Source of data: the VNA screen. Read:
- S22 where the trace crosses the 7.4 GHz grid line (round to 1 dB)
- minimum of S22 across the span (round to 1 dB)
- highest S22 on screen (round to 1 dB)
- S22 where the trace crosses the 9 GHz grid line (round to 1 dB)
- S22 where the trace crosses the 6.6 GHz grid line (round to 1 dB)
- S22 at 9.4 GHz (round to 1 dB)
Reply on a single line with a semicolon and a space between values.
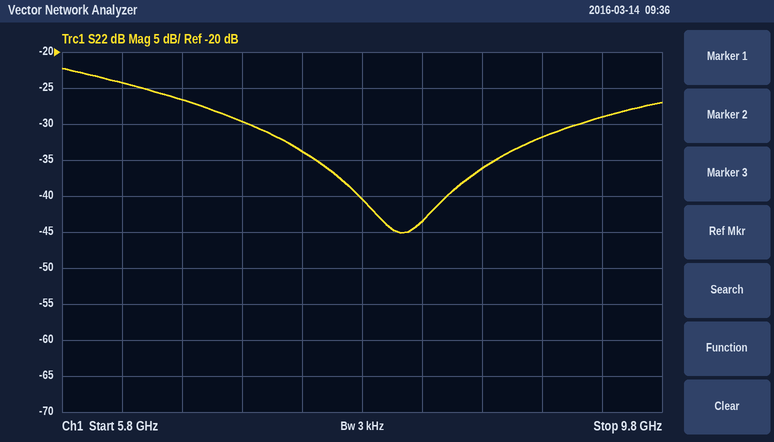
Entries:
-34 dB; -45 dB; -22 dB; -32 dB; -27 dB; -29 dB
